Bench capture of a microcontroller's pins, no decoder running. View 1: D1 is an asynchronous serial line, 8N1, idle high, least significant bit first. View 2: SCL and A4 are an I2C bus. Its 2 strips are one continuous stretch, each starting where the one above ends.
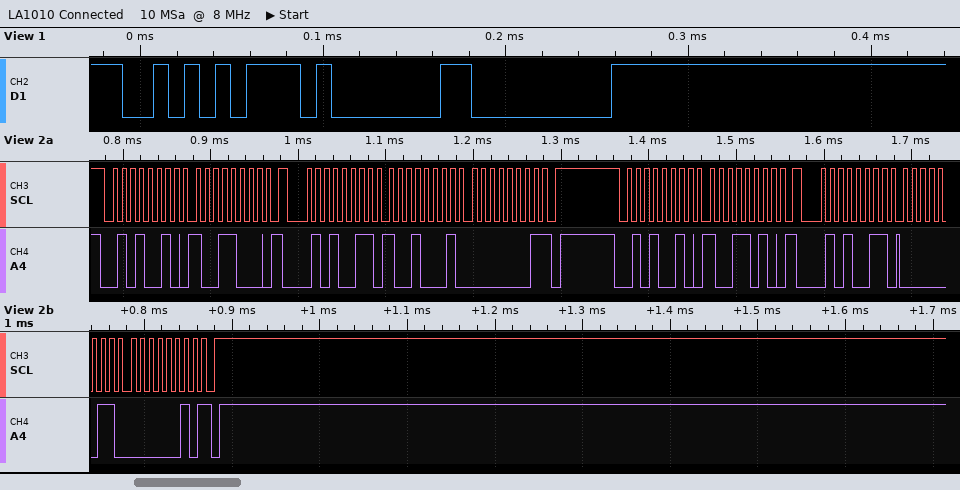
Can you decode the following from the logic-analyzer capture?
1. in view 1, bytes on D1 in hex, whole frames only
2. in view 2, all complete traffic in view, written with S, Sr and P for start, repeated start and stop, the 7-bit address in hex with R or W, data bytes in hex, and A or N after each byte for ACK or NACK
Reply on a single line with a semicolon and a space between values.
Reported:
AA 01 00; S 29W A 98 A Sr 29R A 91 A 01 N P S 29W A 9A A Sr 29R A 03 A 02 N P
